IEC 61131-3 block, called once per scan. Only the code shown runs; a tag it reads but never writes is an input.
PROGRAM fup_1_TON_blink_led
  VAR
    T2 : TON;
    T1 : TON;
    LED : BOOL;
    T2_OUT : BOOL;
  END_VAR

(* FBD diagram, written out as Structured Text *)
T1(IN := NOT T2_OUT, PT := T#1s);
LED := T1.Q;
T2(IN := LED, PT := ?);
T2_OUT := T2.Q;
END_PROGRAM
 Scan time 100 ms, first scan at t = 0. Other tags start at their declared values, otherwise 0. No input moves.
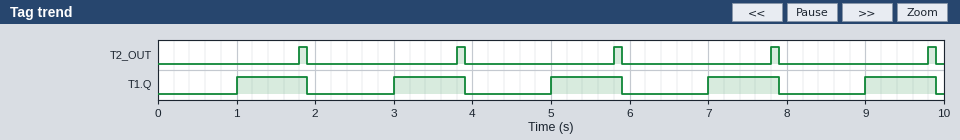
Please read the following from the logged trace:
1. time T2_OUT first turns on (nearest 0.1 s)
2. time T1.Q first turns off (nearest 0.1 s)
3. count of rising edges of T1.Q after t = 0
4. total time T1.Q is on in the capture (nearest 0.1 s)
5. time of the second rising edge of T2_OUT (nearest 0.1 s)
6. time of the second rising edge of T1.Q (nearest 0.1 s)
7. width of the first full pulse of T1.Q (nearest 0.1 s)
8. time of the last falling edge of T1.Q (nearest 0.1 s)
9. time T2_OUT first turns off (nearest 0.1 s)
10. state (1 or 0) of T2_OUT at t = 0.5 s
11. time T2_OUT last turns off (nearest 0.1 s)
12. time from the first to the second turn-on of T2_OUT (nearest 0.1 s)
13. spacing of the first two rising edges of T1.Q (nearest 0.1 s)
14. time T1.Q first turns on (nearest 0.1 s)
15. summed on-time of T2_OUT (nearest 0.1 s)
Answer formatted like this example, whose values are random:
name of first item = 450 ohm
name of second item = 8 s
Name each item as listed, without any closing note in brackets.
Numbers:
time T2_OUT first turns on = 1.8 s
time T1.Q first turns off = 1.9 s
count of rising edges of T1.Q after t = 0 = 5
total time T1.Q is on in the capture = 4.5 s
time of the second rising edge of T2_OUT = 3.8 s
time of the second rising edge of T1.Q = 3.0 s
width of the first full pulse of T1.Q = 0.9 s
time of the last falling edge of T1.Q = 9.9 s
time T2_OUT first turns off = 1.9 s
state (1 or 0) of T2_OUT at t = 0.5 s = 0
time T2_OUT last turns off = 9.9 s
time from the first to the second turn-on of T2_OUT = 2.0 s
spacing of the first two rising edges of T1.Q = 2.0 s
time T1.Q first turns on = 1.0 s
summed on-time of T2_OUT = 0.5 s
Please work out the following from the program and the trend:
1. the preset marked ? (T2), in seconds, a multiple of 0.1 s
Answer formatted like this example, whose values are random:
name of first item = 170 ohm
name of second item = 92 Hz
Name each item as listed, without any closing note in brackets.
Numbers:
the preset marked ? (T2), in seconds, a multiple of 0.1 s = 0.8 s
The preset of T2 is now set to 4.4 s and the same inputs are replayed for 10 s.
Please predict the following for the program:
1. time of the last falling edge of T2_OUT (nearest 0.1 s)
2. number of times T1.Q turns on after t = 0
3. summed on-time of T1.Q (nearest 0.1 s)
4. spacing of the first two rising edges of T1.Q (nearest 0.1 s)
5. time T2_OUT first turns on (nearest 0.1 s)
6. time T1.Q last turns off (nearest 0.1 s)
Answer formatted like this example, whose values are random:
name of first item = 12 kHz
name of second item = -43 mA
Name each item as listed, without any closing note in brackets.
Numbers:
time of the last falling edge of T2_OUT = 5.5 s
number of times T1.Q turns on after t = 0 = 2
summed on-time of T1.Q = 7.9 s
spacing of the first two rising edges of T1.Q = 5.6 s
time T2_OUT first turns on = 5.4 s
time T1.Q last turns off = 5.5 s
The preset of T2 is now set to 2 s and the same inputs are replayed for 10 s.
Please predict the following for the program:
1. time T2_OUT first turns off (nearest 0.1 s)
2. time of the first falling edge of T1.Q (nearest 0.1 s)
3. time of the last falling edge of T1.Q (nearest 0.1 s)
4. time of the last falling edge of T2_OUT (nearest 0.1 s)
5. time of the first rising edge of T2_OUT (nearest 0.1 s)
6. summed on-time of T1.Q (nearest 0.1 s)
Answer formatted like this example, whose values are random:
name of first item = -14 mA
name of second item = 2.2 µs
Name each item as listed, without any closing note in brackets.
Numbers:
time T2_OUT first turns off = 3.1 s
time of the first falling edge of T1.Q = 3.1 s
time of the last falling edge of T1.Q = 9.5 s
time of the last falling edge of T2_OUT = 9.5 s
time of the first rising edge of T2_OUT = 3.0 s
summed on-time of T1.Q = 6.3 s
